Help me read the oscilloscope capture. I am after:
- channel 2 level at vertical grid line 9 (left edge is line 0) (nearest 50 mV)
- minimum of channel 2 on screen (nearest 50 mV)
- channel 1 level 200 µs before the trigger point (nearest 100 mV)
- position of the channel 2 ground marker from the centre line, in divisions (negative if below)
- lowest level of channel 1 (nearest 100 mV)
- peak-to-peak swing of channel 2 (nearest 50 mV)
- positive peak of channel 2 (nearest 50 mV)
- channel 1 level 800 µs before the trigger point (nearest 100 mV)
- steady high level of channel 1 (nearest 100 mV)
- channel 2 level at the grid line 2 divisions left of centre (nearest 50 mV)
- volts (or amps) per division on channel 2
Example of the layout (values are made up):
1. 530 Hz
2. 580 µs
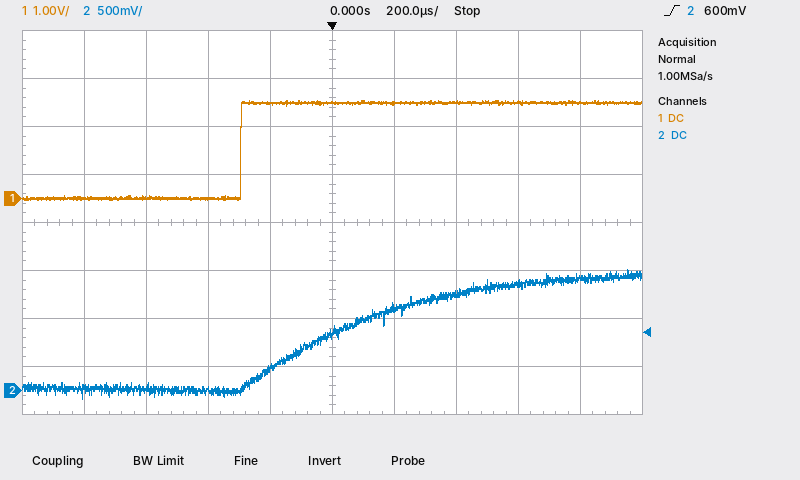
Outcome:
1. 1.15 V
2. -100 mV
3. 2.0 V
4. -3.5 div
5. 0.0 V
6. 1.35 V
7. 1.25 V
8. 0.0 V
9. 2.0 V
10. 0 mV
11. 500 mV
